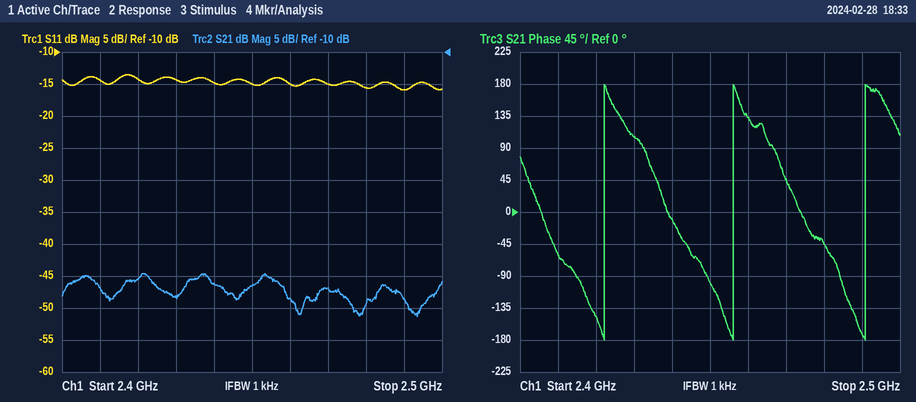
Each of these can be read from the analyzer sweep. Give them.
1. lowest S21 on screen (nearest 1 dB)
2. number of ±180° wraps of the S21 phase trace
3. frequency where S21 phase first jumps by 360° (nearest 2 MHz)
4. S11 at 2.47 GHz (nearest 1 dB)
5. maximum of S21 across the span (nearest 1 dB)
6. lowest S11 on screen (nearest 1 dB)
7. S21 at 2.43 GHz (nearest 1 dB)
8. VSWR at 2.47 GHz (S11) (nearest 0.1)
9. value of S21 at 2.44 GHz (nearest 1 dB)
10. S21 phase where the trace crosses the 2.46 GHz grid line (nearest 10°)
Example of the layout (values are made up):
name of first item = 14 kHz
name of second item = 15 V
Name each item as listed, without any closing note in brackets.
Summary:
lowest S21 on screen = -51 dB
number of ±180° wraps of the S21 phase trace = 3
frequency where S21 phase first jumps by 360° = 2.422 GHz
S11 at 2.47 GHz = -15 dB
maximum of S21 across the span = -45 dB
lowest S11 on screen = -16 dB
S21 at 2.43 GHz = -48 dB
VSWR at 2.47 GHz (S11) = 1.4
value of S21 at 2.44 GHz = -46 dB
S21 phase where the trace crosses the 2.46 GHz grid line = 130°
